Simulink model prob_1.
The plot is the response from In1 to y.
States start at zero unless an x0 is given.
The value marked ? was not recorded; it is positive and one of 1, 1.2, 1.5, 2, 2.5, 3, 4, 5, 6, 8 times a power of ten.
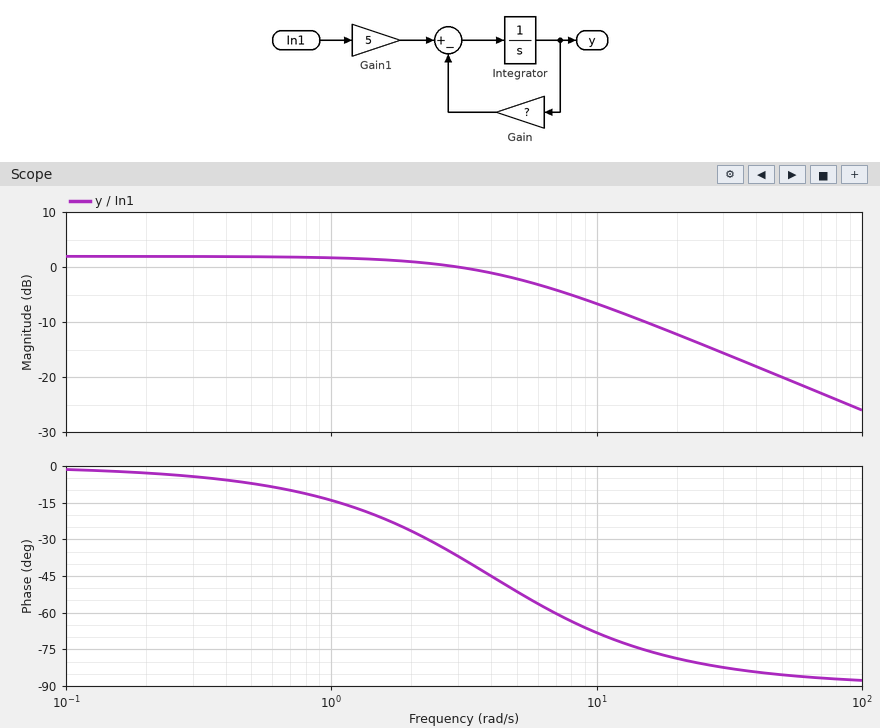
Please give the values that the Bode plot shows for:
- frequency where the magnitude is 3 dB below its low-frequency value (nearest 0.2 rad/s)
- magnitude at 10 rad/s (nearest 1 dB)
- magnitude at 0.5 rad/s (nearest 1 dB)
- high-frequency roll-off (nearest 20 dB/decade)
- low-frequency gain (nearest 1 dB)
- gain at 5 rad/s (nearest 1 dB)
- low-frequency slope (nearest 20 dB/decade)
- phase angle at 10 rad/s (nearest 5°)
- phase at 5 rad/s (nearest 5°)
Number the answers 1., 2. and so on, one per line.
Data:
1. 4.0 rad/s
2. -7 dB
3. 2 dB
4. -20 dB/decade
5. 2 dB
6. -2 dB
7. 0 dB/decade
8. -70°
9. -50°
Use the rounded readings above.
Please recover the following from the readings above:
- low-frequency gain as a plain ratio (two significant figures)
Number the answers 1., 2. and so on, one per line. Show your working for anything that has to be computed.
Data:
1. 10^(2 / 20) = 1.3
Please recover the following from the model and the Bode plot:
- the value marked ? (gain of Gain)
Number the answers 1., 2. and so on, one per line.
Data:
1. 4
